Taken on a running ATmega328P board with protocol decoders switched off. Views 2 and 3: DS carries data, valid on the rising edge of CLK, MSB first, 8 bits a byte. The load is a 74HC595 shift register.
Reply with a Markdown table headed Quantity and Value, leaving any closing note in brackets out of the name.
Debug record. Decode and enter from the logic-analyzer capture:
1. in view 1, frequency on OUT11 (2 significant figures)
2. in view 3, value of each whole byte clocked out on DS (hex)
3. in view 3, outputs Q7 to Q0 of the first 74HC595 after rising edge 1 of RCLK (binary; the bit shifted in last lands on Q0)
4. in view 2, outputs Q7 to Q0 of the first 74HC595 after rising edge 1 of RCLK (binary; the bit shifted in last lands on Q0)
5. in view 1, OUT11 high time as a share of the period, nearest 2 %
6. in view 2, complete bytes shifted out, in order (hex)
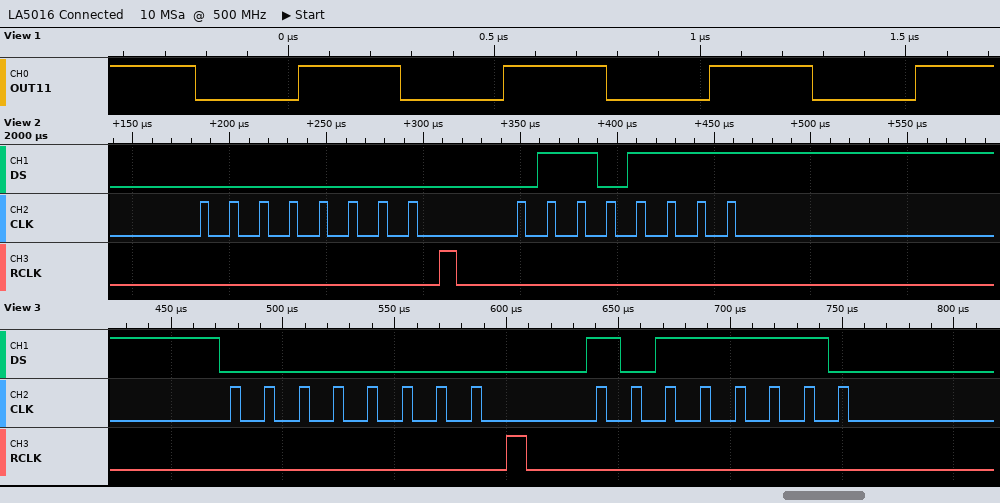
| Quantity | Value |
|---|---|
| in view 1, frequency on OUT11 | 2.0 MHz |
| in view 3, value of each whole byte clocked out on DS | 00 BE |
| in view 3, outputs Q7 to Q0 of the first 74HC595 after rising edge 1 of RCLK | 00000000 |
| in view 2, outputs Q7 to Q0 of the first 74HC595 after rising edge 1 of RCLK | 00000000 |
| in view 1, OUT11 high time as a share of the period, nearest 2 % | 50 % |
| in view 2, complete bytes shifted out, in order | 0x00 0x6F |
